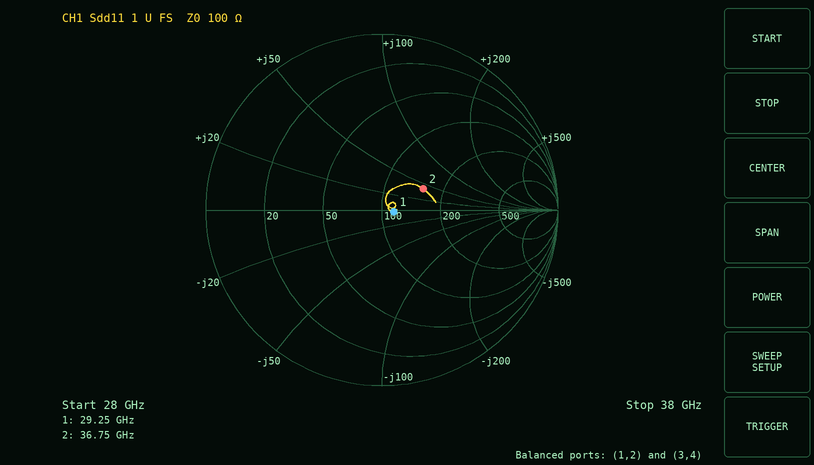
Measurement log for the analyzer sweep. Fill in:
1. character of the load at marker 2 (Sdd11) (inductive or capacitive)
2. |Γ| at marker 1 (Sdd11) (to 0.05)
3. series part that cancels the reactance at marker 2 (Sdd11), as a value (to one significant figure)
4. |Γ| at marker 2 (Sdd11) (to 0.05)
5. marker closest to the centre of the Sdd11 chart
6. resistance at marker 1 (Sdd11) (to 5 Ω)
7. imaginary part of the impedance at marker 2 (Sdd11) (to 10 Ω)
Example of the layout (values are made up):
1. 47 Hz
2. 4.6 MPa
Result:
1. inductive
2. 0.05
3. 100 fF
4. 0.25
5. marker 1
6. 115 Ω
7. +40 Ω
